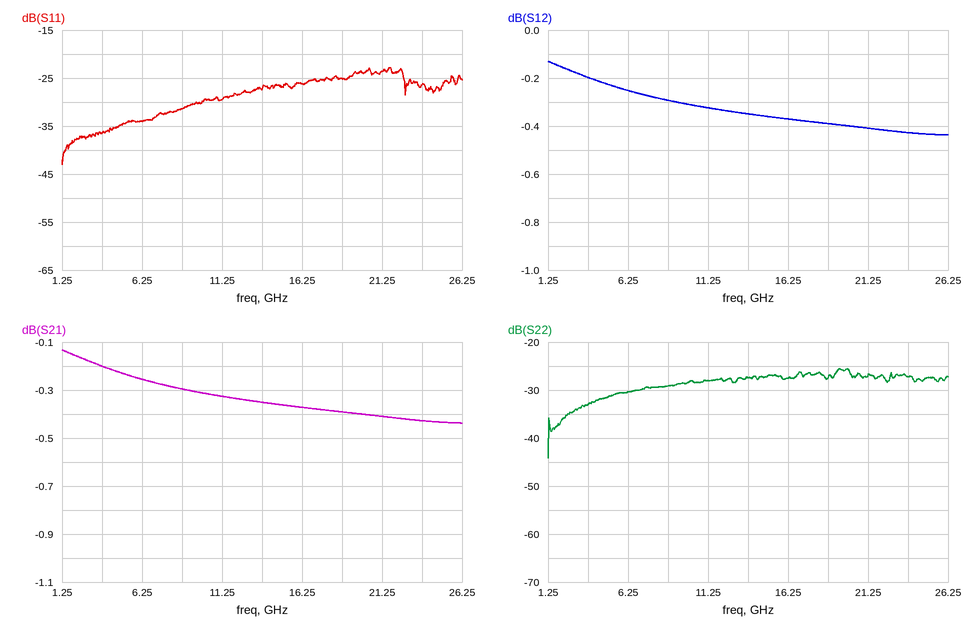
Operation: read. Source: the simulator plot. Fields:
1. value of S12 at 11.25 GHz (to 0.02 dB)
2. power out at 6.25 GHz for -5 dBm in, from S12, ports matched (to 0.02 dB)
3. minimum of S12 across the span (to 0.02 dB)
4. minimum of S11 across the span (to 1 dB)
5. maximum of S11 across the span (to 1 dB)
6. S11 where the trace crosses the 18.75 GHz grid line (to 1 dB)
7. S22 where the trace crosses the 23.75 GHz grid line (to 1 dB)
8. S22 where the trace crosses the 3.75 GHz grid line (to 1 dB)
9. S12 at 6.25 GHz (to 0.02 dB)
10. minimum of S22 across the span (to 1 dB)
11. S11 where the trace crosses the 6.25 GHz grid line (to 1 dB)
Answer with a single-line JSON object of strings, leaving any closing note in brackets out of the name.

{"value of S12 at 11.25 GHz": "-0.32 dB", "power out at 6.25 GHz for -5 dBm in, from S12, ports matched": "-5.26 dBm", "minimum of S12 across the span": "-0.44 dB", "minimum of S11 across the span": "-43 dB", "maximum of S11 across the span": "-23 dB", "S11 where the trace crosses the 18.75 GHz grid line": "-25 dB", "S22 where the trace crosses the 23.75 GHz grid line": "-27 dB", "S22 where the trace crosses the 3.75 GHz grid line": "-33 dB", "S12 at 6.25 GHz": "-0.26 dB", "minimum of S22 across the span": "-44 dB", "S11 where the trace crosses the 6.25 GHz grid line": "-34 dB"}
